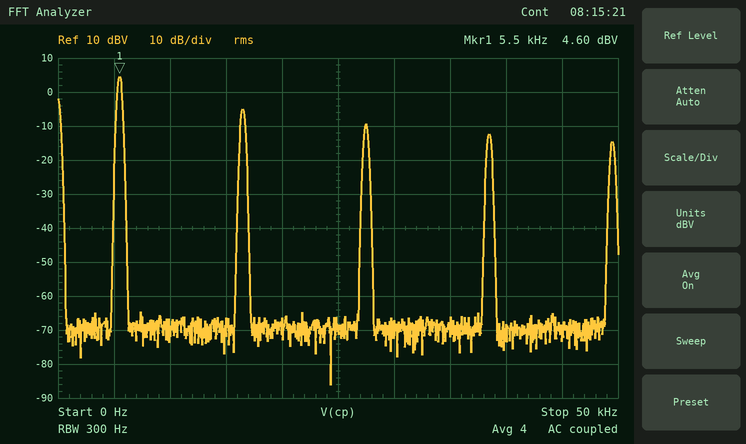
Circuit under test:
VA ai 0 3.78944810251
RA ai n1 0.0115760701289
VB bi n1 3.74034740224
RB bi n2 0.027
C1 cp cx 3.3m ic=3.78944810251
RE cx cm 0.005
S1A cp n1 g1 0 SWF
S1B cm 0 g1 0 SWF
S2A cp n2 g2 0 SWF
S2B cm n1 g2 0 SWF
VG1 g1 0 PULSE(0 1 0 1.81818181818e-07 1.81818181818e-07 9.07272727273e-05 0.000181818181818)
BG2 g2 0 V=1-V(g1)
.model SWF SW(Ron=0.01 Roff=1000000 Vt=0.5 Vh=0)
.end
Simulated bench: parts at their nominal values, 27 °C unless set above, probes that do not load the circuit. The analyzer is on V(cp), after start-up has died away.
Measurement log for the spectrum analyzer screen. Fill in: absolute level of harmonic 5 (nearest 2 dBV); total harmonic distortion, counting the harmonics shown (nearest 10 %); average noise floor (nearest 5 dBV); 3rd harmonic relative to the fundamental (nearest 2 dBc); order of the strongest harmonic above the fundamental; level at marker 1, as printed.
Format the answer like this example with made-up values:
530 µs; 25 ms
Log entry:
-10 dBV; 40 %; -70 dBV; -10 dBc; 3; 4.60 dBV
